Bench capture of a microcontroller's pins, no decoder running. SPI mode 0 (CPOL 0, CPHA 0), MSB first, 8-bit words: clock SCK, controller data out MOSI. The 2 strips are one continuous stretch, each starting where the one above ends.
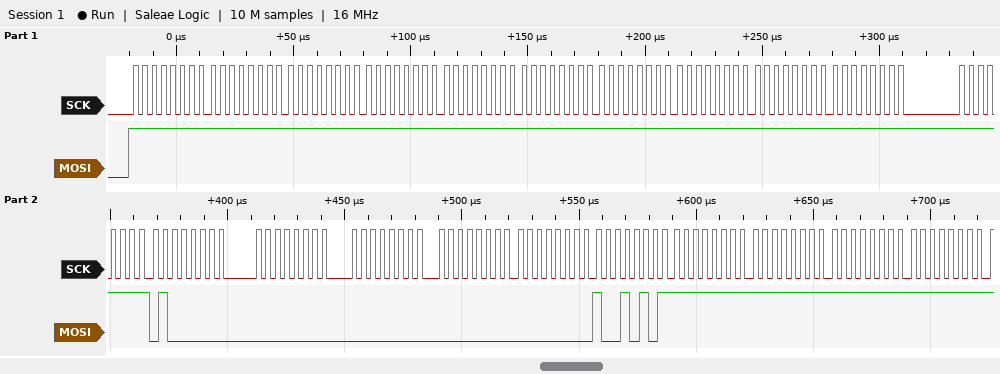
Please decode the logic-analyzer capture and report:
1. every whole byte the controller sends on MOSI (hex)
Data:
0xFF 0xFF 0xFF 0xFF 0xFF 0xFF 0xFF 0xFF 0xFF 0xFF 0xFF 0x40 0x00 0x00 0x00 0x00 0x95 0xFF 0xFF 0xFF 0xFF
